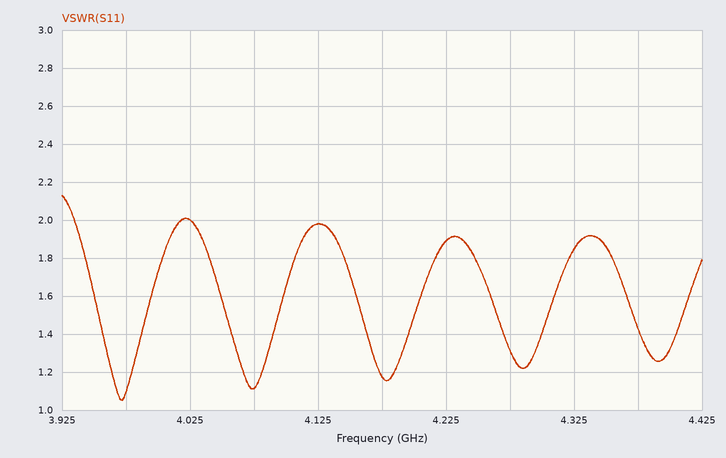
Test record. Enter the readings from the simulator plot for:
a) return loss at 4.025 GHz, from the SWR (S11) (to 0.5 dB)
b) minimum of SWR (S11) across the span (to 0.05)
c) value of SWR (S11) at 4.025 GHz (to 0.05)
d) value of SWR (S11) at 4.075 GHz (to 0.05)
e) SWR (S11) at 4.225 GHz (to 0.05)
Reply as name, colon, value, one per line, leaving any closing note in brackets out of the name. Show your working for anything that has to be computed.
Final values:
return loss at 4.025 GHz, from the SWR (S11): −20 log10((2 − 1)/(2 + 1)) ≈ 9.5 dB
minimum of SWR (S11) across the span: 1.05
value of SWR (S11) at 4.025 GHz: 2.00
value of SWR (S11) at 4.075 GHz: 1.10
SWR (S11) at 4.225 GHz: 1.90
